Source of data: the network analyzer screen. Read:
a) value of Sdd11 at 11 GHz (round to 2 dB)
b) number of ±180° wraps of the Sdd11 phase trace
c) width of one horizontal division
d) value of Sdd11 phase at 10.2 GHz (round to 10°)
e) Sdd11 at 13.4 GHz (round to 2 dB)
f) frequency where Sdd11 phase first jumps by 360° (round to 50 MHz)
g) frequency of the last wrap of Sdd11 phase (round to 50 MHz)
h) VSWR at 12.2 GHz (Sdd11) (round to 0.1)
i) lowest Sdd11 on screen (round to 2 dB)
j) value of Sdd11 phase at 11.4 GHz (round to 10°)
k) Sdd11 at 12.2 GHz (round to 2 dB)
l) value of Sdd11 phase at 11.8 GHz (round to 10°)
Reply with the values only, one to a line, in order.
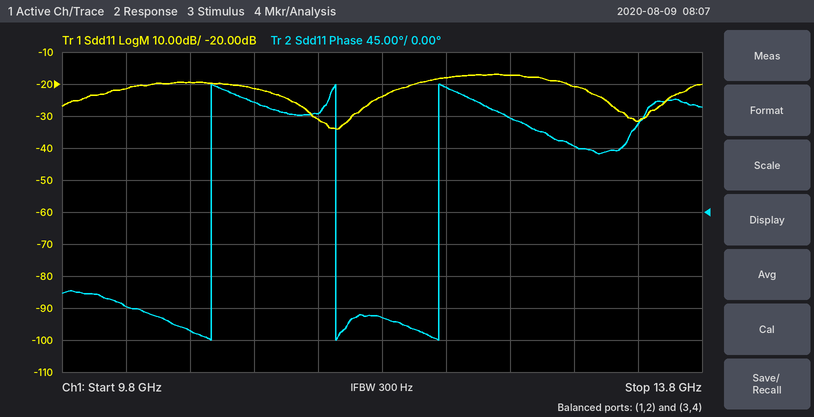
-22 dB
3
400 MHz
-130°
-32 dB
10.75 GHz
12.15 GHz
1.3
-34 dB
140°
-18 dB
-150°
